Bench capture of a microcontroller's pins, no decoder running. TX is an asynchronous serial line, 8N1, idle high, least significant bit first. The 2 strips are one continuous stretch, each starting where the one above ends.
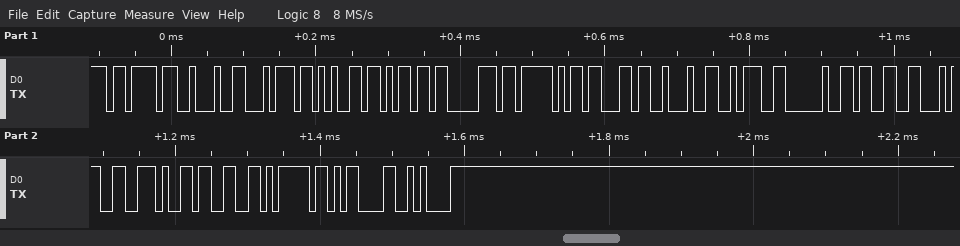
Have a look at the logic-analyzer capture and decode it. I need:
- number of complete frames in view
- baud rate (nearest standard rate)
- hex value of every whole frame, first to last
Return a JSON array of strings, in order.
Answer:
["18", "115200 baud", "7B 22 74 65 6D 70 5F 63 22 3A 20 33 34 2E 33 7D 0D 0A"]
